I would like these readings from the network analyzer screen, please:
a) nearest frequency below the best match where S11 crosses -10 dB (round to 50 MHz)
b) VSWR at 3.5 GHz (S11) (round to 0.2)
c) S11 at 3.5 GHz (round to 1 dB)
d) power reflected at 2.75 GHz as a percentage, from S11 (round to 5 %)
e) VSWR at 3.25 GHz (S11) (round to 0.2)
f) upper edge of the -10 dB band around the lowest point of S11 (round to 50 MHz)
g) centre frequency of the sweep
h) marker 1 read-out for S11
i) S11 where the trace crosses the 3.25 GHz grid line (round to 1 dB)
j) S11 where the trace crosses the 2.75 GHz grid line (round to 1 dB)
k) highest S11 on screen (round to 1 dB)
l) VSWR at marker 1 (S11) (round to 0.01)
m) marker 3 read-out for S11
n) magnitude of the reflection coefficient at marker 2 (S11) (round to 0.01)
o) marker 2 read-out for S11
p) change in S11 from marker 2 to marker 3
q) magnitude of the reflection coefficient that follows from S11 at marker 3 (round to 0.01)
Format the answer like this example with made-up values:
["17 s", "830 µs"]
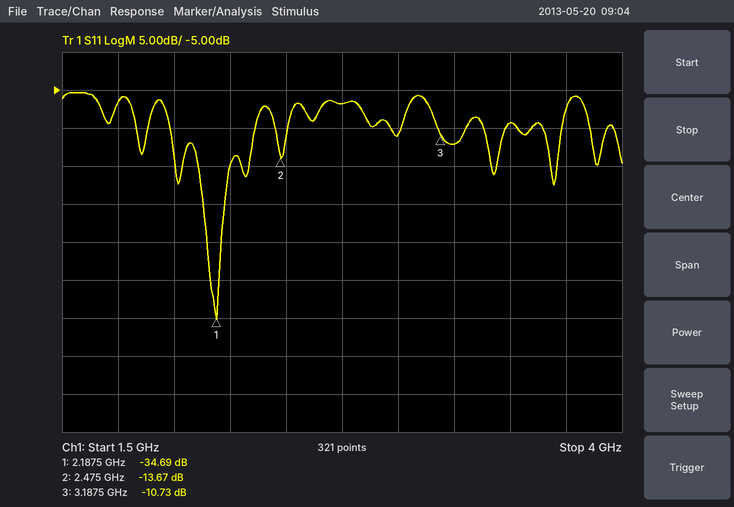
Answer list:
["2.00 GHz", "2.0", "-9 dB", "20 %", "1.6", "2.35 GHz", "2.75 GHz", "-34.69 dB", "-12 dB", "-7 dB", "-5 dB", "1.04", "-10.73 dB", "0.21", "-13.67 dB", "2.94 dB", "0.29"]
